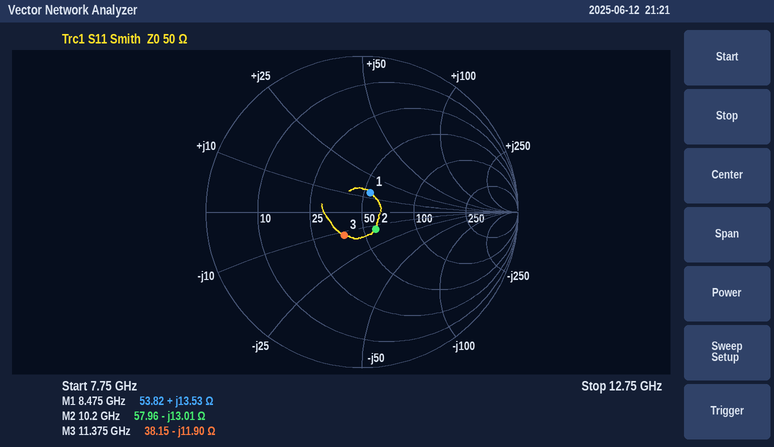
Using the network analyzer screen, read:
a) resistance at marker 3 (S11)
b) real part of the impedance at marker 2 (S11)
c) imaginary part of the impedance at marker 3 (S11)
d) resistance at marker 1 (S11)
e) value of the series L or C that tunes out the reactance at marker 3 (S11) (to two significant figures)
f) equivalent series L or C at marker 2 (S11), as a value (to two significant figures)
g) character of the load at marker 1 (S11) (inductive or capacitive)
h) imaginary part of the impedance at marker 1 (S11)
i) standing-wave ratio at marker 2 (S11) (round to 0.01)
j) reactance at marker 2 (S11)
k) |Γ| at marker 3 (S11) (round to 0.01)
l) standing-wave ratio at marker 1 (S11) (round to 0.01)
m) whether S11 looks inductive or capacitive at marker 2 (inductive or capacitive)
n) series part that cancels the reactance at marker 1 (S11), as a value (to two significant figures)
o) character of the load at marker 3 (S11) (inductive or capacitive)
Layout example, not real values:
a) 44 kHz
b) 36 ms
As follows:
a) 38.15 Ω
b) 57.96 Ω
c) -11.90 Ω
d) 53.82 Ω
e) 170 pH
f) 1.2 pF
g) inductive
h) +13.53 Ω
i) 1.33
j) -13.01 Ω
k) 0.19
l) 1.31
m) capacitive
n) 1.4 pF
o) capacitive
